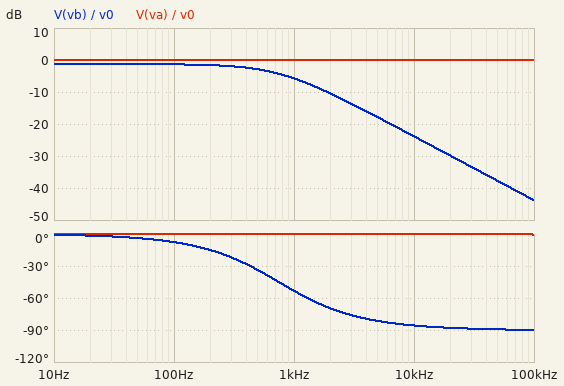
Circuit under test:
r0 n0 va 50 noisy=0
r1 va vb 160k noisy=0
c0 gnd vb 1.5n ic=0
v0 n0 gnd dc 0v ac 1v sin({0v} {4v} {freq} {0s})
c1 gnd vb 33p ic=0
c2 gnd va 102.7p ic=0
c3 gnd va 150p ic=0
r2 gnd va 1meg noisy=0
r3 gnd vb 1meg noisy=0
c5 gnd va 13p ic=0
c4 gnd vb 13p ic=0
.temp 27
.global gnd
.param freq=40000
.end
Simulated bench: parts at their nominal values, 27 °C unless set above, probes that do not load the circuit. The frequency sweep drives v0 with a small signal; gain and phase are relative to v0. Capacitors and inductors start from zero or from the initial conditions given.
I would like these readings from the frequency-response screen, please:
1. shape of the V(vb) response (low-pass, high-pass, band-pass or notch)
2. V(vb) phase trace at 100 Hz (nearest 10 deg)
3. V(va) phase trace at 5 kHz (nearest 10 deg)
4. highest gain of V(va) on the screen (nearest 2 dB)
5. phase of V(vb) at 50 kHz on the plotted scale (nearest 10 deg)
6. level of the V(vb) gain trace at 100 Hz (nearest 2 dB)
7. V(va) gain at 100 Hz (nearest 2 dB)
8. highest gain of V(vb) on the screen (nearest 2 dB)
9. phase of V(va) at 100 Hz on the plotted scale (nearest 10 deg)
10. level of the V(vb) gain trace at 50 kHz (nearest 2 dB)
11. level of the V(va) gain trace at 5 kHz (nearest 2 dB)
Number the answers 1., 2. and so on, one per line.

1. low-pass
2. -10 deg
3. 0 deg
4. 0 dB
5. -90 deg
6. -2 dB
7. 0 dB
8. -2 dB
9. 0 deg
10. -38 dB
11. 0 dB
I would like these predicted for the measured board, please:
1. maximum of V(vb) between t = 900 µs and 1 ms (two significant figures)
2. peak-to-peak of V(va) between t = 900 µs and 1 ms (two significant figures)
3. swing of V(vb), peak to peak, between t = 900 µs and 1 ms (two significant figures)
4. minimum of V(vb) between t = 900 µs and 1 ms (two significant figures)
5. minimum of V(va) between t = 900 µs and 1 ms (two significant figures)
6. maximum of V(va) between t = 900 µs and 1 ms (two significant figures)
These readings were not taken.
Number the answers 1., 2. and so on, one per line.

1. 65 mV
2. 8.0 V
3. 130 mV
4. -64 mV
5. -4.0 V
6. 4.0 V
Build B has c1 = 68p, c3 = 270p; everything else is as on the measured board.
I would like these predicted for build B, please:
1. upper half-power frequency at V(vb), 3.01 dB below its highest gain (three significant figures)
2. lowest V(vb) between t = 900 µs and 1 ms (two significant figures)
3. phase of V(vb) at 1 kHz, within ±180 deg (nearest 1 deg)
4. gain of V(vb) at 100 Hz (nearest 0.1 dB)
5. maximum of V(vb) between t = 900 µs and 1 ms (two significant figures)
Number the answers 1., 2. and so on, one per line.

1. 730 Hz
2. -62 mV
3. -54 deg
4. -1.4 dB
5. 64 mV
